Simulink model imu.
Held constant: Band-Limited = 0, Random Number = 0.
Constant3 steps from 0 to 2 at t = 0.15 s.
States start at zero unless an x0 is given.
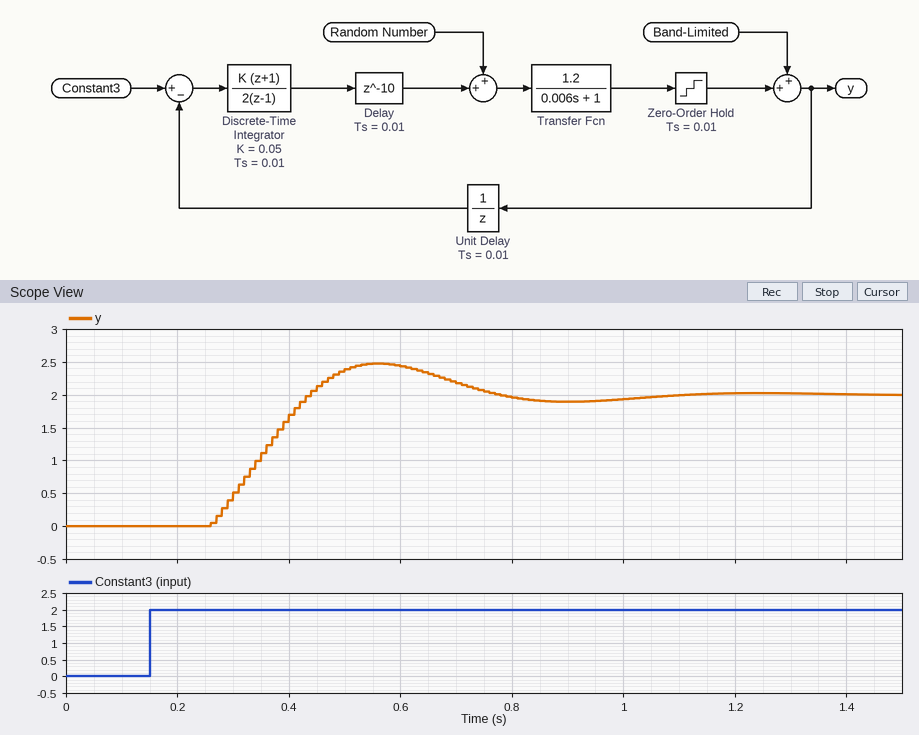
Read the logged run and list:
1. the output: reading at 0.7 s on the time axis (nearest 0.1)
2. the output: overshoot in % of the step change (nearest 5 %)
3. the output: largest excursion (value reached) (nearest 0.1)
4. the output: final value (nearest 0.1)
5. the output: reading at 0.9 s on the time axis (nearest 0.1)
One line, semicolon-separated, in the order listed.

2.2; 25 %; 2.5; 2.0; 1.9
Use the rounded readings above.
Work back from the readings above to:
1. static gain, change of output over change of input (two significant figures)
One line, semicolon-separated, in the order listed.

1.0
